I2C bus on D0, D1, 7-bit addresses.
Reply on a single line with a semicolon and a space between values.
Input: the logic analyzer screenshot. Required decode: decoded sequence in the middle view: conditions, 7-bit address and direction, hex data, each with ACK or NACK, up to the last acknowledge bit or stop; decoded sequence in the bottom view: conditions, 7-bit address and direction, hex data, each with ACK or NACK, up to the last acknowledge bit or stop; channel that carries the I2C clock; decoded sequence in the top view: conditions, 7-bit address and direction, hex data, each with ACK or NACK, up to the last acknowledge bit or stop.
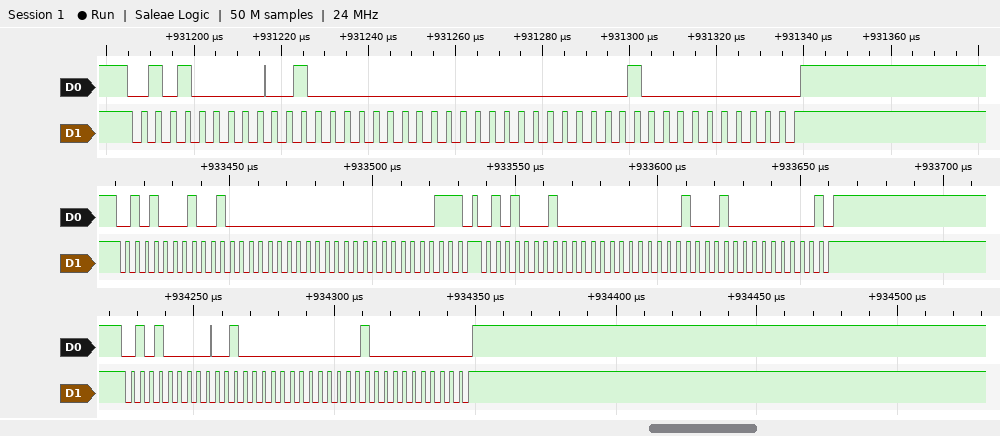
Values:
start, address 28 read ACK, 40 ACK, 00 ACK, 03 NACK, stop, start, address 28 read ACK, 00 ACK, 11 ACK, 00 NACK, stop; start, address 28 write ACK, 20 ACK, 01 ACK, 00 ACK, stop; D1; start, address 28 write ACK, 20 ACK, 00 ACK, 01 ACK, 00 ACK, stop
